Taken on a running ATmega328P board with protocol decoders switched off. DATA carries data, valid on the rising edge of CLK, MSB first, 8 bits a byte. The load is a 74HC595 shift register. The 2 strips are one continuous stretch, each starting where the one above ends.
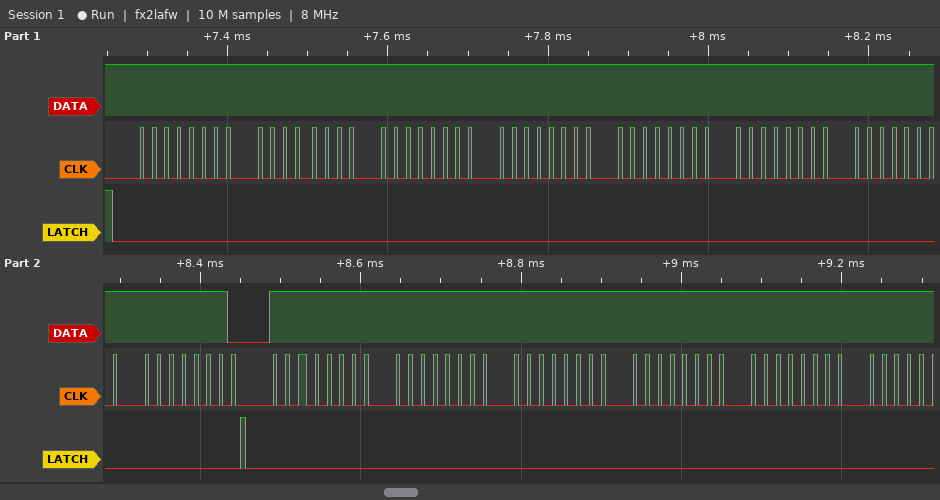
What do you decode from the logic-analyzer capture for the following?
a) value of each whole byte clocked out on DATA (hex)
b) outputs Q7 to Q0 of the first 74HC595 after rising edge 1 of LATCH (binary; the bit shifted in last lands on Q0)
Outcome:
0xFF 0xFF 0xFF 0xFF 0xFF 0xFF 0xFF 0xFE 0xFF 0xFF 0xFF 0xFF 0xFF
11111110
